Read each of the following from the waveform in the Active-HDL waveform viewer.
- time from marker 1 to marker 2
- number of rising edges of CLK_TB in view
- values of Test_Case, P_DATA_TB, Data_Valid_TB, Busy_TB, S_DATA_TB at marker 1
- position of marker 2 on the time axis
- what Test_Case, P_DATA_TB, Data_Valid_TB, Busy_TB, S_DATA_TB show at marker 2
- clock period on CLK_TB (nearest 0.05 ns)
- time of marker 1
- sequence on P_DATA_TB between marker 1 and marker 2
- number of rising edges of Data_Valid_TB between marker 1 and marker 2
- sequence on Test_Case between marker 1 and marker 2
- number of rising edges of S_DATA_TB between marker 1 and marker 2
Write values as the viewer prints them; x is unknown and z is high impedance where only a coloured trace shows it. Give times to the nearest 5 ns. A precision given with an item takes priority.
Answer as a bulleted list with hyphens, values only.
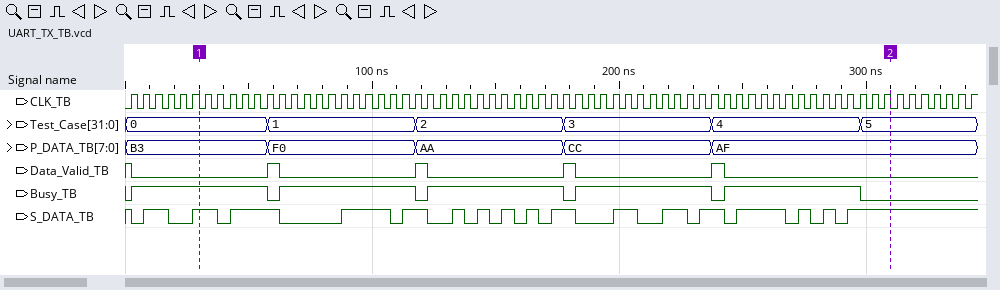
- 280 ns
- 69
- Test_Case=0, P_DATA_TB=B3, Data_Valid_TB=0, Busy_TB=1, S_DATA_TB=1
- 310 ns
- Test_Case=5, P_DATA_TB=AF, Data_Valid_TB=0, Busy_TB=0, S_DATA_TB=1
- 5 ns
- 30 ns
- B3, F0, AA, CC, AF
- 4
- 0, 1, 2, 3, 4, 5
- 15
